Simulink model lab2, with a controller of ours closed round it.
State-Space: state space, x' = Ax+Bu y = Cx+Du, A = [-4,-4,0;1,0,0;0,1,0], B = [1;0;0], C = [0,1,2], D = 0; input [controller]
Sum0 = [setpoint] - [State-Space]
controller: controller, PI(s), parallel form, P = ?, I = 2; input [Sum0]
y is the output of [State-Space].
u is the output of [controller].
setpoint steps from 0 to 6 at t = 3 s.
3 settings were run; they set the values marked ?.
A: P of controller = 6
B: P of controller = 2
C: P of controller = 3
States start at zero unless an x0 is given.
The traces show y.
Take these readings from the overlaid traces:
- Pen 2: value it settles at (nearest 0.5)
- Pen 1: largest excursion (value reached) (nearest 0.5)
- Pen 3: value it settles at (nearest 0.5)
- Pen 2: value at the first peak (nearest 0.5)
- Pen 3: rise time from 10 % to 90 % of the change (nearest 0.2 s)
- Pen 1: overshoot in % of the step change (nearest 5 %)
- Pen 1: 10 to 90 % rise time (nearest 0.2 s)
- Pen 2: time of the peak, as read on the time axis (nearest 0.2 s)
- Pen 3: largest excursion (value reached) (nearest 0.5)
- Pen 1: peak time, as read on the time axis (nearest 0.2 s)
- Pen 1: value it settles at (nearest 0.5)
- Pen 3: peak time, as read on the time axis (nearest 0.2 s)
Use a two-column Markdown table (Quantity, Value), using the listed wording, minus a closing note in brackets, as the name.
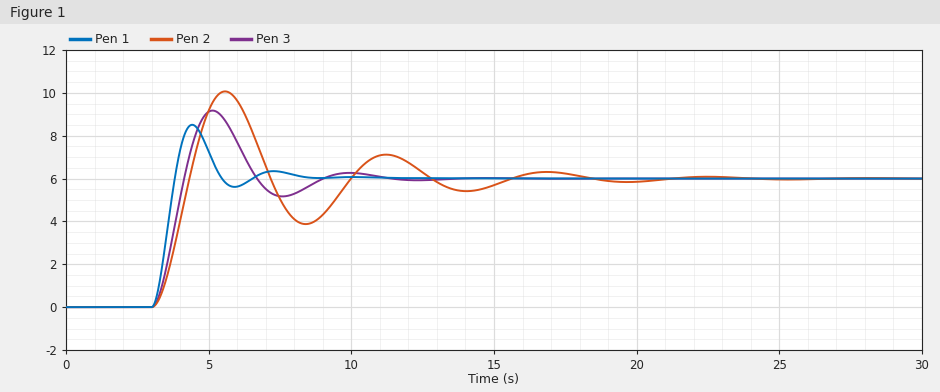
| Quantity | Value |
|---|---|
| Pen 2: value it settles at | 6.0 |
| Pen 1: largest excursion (value reached) | 8.5 |
| Pen 3: value it settles at | 6.0 |
| Pen 2: value at the first peak | 10.0 |
| Pen 3: rise time from 10 % to 90 % of the change | 0.8 s |
| Pen 1: overshoot in % of the step change | 40 % |
| Pen 1: 10 to 90 % rise time | 0.6 s |
| Pen 2: time of the peak, as read on the time axis | 5.6 s |
| Pen 3: largest excursion (value reached) | 9.0 |
| Pen 1: peak time, as read on the time axis | 4.4 s |
| Pen 1: value it settles at | 6.0 |
| Pen 3: peak time, as read on the time axis | 5.2 s |
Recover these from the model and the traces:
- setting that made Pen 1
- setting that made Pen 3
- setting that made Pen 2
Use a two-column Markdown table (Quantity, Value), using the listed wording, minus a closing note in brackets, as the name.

| Quantity | Value |
|---|---|
| setting that made Pen 1 | A |
| setting that made Pen 3 | C |
| setting that made Pen 2 | B |
